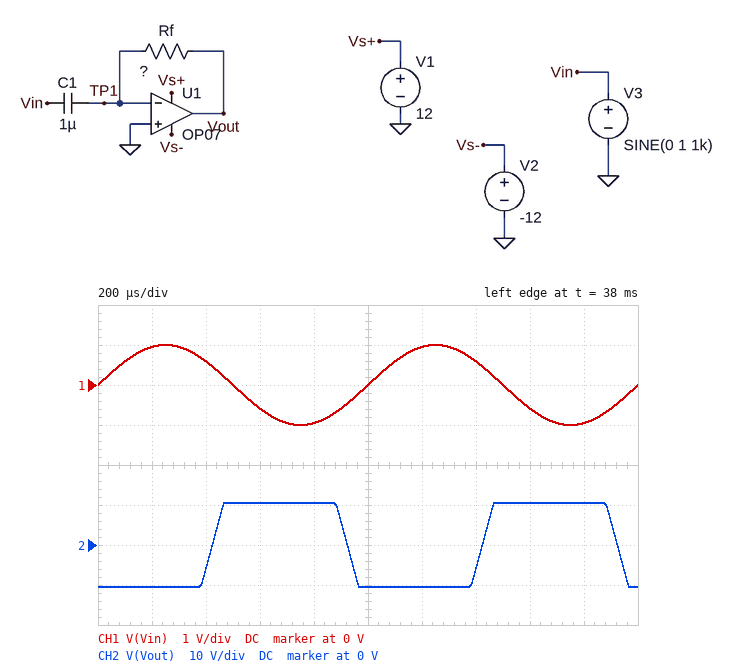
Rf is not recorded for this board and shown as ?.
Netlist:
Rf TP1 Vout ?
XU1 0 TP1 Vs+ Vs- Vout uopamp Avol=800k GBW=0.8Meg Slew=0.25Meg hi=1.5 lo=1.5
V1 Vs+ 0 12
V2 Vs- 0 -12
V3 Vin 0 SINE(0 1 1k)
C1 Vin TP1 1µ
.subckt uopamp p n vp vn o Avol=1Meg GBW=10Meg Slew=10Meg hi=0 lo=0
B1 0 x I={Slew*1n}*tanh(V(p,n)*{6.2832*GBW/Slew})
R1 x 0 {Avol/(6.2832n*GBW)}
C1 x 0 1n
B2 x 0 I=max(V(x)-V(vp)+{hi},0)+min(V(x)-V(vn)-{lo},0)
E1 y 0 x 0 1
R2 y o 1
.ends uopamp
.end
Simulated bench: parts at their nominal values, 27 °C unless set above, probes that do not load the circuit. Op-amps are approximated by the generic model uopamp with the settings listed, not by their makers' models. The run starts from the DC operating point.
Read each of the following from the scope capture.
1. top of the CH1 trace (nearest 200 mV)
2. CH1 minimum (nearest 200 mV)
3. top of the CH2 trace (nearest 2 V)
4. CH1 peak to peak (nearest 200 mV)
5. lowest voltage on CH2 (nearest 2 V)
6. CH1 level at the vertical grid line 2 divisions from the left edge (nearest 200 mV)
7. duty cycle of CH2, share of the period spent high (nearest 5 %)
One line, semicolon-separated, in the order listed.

1.0 V; -1.0 V; 10 V; 2.0 V; -10 V; 600 mV; 50 %
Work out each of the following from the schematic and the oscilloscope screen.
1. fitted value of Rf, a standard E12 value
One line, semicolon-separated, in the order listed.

3.3 kΩ
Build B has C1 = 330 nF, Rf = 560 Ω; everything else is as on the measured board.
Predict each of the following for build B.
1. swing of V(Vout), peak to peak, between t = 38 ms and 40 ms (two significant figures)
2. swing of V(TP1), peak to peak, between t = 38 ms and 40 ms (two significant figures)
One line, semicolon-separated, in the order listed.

2.3 V; 2.9 mV
